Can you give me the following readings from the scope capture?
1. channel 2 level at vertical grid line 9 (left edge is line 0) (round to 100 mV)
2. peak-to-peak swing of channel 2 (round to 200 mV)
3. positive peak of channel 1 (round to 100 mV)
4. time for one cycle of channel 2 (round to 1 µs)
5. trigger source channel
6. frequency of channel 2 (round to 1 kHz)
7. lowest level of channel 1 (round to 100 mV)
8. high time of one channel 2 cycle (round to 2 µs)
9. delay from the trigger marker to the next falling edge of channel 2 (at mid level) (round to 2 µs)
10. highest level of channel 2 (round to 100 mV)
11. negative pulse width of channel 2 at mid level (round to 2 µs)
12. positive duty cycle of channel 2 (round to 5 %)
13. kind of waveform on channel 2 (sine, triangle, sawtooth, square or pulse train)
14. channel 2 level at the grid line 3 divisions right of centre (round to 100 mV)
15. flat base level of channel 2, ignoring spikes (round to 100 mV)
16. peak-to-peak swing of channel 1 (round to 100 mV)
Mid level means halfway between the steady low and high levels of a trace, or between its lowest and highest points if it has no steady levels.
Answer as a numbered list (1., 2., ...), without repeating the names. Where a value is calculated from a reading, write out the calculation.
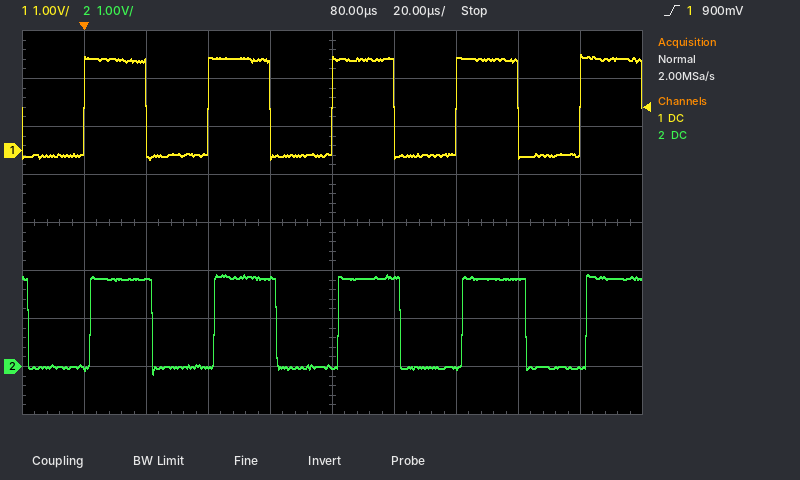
1. 0.0 V
2. 2.0 V
3. 2.0 V
4. 40 µs
5. channel 1
6. 1 / 40 µs ≈ 25 kHz
7. -200 mV
8. 20 µs
9. 22 µs
10. 1.9 V
11. 20 µs
12. 20 µs / 40 µs ≈ 50 %
13. square
14. 1.8 V
15. 0.0 V
16. 2.0 V − (-200 mV) = 2.2 V
